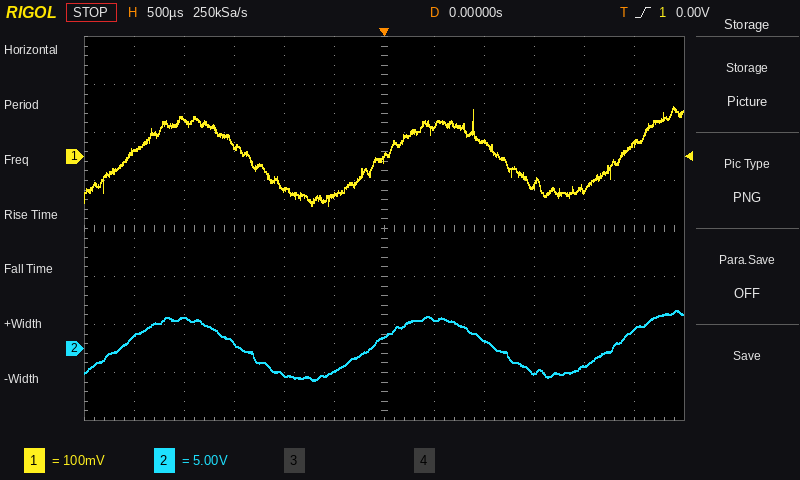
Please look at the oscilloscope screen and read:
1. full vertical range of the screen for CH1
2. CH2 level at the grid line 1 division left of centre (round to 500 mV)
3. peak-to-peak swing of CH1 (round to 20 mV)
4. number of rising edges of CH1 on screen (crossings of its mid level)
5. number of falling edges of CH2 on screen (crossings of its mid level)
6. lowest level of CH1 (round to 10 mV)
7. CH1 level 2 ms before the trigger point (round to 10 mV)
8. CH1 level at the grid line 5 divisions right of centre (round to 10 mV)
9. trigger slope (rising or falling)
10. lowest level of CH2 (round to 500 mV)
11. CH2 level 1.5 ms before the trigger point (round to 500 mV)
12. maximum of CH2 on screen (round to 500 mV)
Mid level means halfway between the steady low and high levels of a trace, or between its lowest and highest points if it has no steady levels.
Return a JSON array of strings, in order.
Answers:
["800 mV", "-2.5 V", "200 mV", "3", "2", "-100 mV", "80 mV", "30 mV", "rising", "-3.5 V", "500 mV", "4.0 V"]
